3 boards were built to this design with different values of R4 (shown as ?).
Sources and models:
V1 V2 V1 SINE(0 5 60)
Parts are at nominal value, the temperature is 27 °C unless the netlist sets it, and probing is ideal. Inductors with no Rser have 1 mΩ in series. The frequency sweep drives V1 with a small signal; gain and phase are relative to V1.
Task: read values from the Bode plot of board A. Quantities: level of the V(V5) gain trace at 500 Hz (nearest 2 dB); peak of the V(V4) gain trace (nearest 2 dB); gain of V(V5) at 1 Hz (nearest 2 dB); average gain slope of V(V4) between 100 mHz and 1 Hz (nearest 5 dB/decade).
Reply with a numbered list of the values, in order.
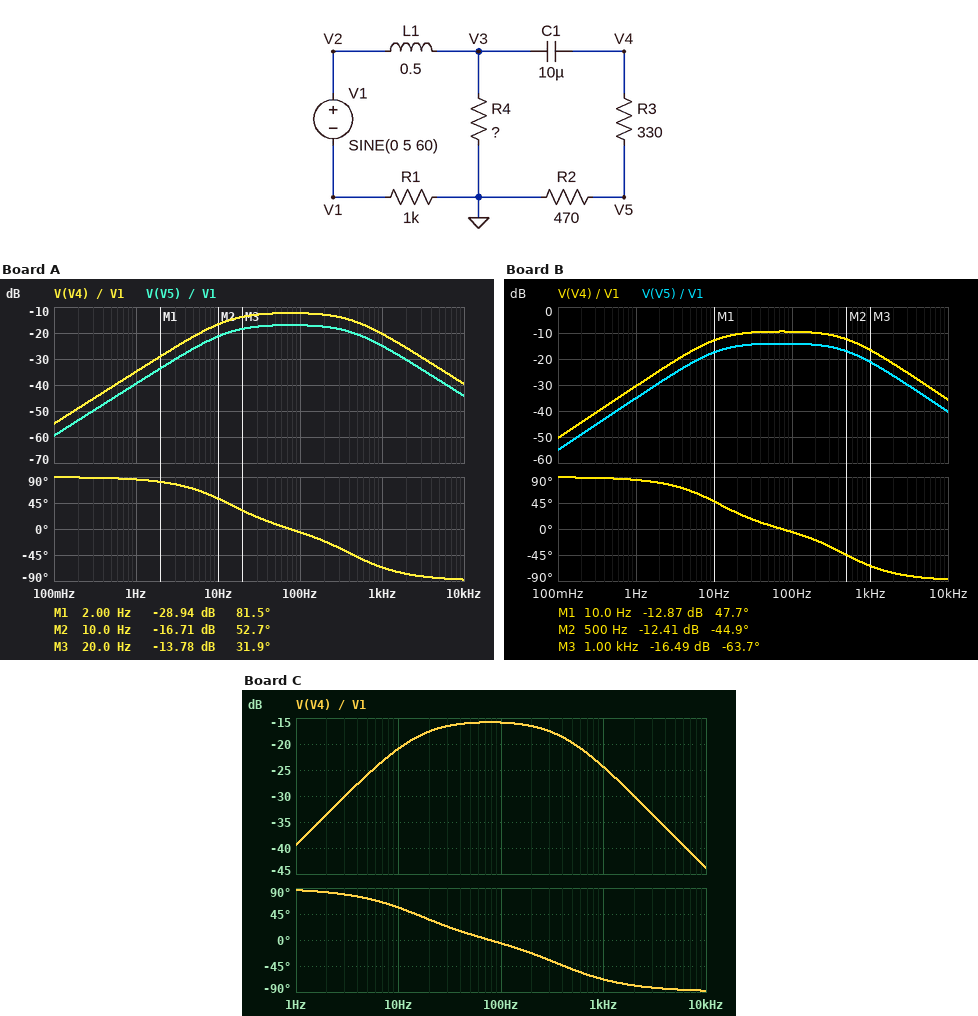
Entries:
1. -20 dB
2. -12 dB
3. -40 dB
4. 20 dB/decade
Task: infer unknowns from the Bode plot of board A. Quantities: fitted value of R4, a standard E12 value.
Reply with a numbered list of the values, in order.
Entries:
1. 560 Ω
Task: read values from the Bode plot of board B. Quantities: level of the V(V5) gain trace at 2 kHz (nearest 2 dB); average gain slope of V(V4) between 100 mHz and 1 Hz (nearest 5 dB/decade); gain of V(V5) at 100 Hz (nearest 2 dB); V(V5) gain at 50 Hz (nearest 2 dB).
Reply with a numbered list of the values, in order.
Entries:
1. -26 dB
2. 20 dB/decade
3. -14 dB
4. -14 dB
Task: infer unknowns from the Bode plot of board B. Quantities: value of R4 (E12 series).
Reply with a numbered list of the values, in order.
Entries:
1. 1.5 kΩ
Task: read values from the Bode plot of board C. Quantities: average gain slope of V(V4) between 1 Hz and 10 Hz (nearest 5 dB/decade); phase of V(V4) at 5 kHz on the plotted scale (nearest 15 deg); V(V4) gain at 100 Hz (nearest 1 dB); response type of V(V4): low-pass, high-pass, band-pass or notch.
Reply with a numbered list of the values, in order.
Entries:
1. 20 dB/decade
2. -90 deg
3. -16 dB
4. band-pass
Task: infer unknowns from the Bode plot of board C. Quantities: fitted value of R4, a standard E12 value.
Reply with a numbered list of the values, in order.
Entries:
1. 270 Ω
